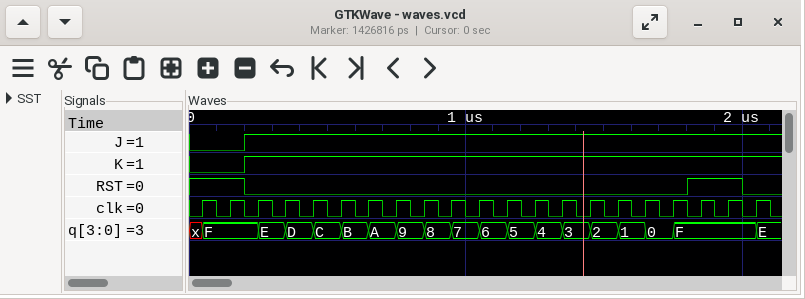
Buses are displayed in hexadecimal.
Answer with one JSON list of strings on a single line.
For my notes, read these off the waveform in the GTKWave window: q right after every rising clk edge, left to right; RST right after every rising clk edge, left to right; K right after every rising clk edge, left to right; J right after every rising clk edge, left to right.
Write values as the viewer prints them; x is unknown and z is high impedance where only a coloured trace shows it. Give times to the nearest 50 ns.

["F, F, E, D, C, B, A, 9, 8, 7, 6, 5, 4, 3, 2, 1, 0, F, F, F, E", "1 1 0 0 0 0 0 0 0 0 0 0 0 0 0 0 0 0 1 1 0", "0 0 1 1 1 1 1 1 1 1 1 1 1 1 1 1 1 1 1 1 1", "0 0 1 1 1 1 1 1 1 1 1 1 1 1 1 1 1 1 1 1 1"]
